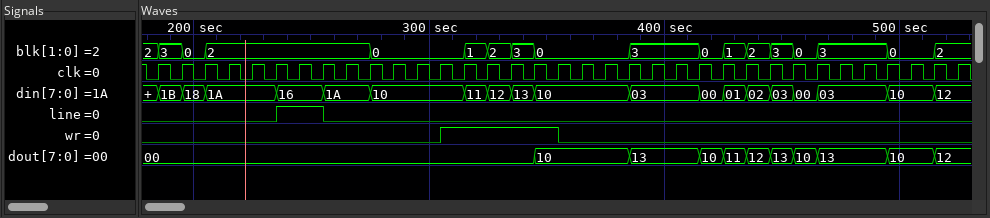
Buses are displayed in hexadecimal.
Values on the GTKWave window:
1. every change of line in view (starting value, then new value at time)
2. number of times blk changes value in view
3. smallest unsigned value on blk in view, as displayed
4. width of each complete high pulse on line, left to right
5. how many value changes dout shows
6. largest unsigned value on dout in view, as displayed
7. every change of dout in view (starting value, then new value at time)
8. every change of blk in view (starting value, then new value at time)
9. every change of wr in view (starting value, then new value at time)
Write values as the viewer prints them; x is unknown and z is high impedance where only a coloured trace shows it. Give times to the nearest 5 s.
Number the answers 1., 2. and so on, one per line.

1. 0, 1 at 235 s, 0 at 255 s
2. 17
3. 0
4. 20 s
5. 10
6. 13
7. 00, 10 at 345 s, 13 at 385 s, 10 at 415 s, 11 at 425 s, 12 at 435 s, 13 at 445 s, 10 at 455 s, 13 at 465 s, 10 at 495 s, 12 at 515 s
8. 2, 3 at 185 s, 0 at 195 s, 2 at 205 s, 0 at 275 s, 1 at 315 s, 2 at 325 s, 3 at 335 s, 0 at 345 s, 3 at 385 s, 0 at 415 s, 1 at 425 s, 2 at 435 s, 3 at 445 s, 0 at 455 s, 3 at 465 s, 0 at 495 s, 2 at 515 s
9. 0, 1 at 305 s, 0 at 355 s
